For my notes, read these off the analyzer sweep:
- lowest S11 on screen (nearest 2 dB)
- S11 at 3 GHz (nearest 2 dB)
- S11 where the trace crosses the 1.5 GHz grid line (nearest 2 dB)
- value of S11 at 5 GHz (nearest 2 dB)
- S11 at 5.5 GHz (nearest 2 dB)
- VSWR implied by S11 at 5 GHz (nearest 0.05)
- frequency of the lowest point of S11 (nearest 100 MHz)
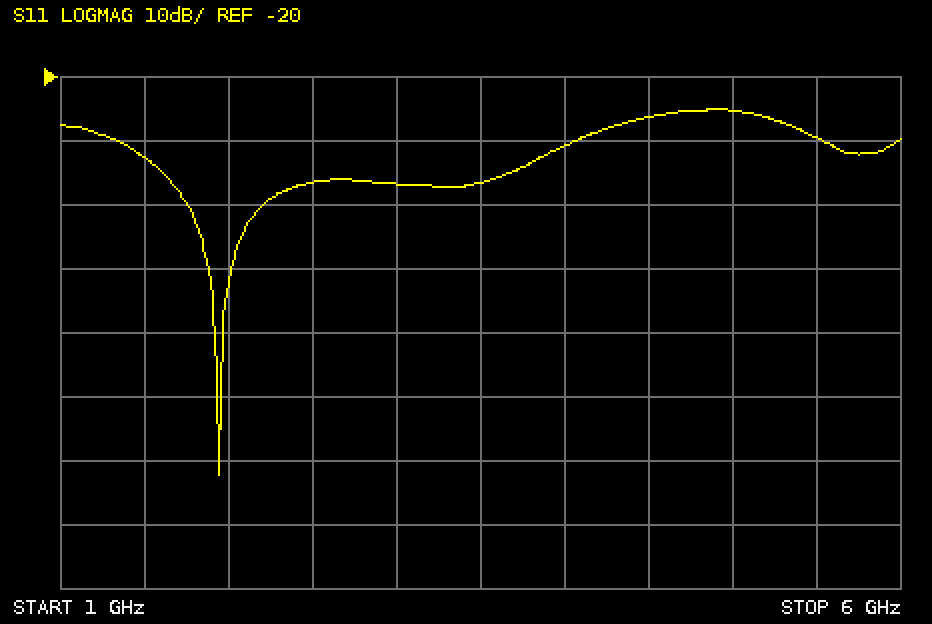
-82 dB
-36 dB
-32 dB
-26 dB
-30 dB
1.10
1.9 GHz
